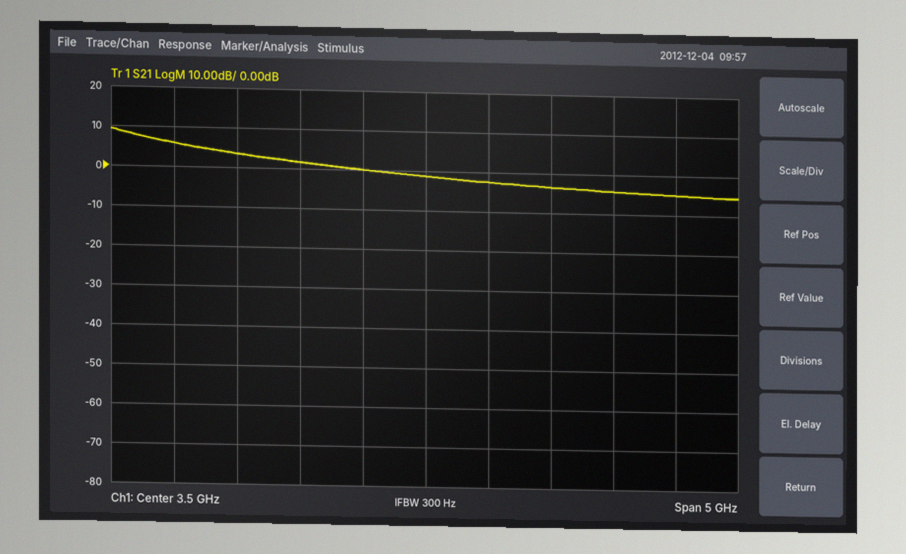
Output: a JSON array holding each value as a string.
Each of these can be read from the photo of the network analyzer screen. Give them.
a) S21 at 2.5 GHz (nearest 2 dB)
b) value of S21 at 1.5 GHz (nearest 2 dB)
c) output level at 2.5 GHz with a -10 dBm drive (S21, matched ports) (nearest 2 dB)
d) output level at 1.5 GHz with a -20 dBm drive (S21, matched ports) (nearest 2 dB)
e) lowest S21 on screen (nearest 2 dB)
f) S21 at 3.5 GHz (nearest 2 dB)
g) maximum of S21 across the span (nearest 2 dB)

["2 dB", "6 dB", "-8 dBm", "-14 dBm", "-6 dB", "-2 dB", "10 dB"]
